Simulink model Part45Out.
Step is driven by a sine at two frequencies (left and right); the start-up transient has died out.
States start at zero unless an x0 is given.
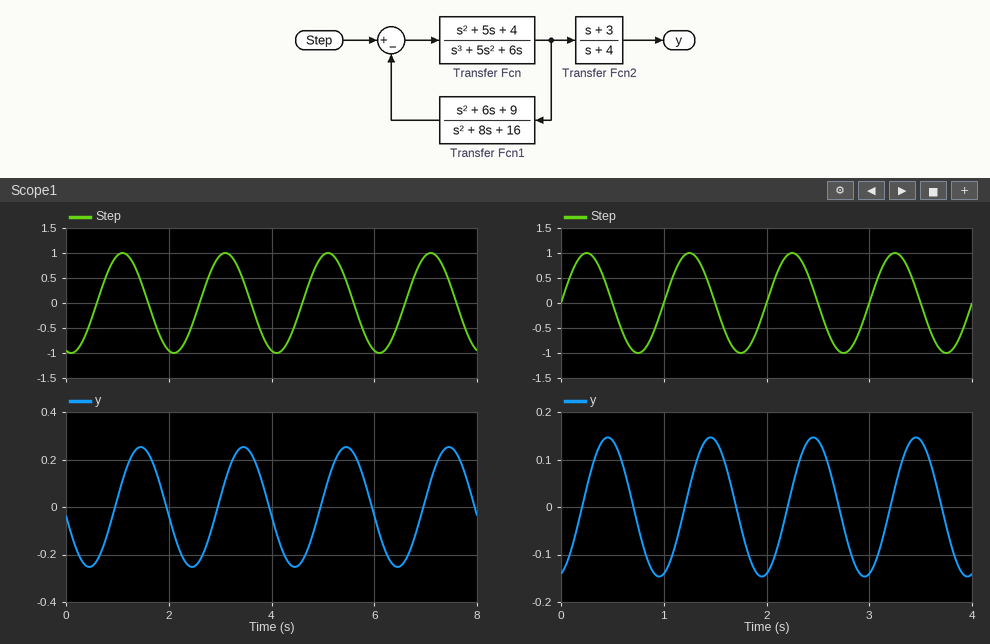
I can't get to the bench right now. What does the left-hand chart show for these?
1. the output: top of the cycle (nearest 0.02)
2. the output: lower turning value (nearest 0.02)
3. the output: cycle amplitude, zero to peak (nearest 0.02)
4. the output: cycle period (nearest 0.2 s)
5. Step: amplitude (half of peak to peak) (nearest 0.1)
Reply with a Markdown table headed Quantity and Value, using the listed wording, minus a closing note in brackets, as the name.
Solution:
| Quantity | Value |
|---|---|
| the output: top of the cycle | 0.26 |
| the output: lower turning value | -0.26 |
| the output: cycle amplitude, zero to peak | 0.26 |
| the output: cycle period | 2.0 s |
| Step: amplitude (half of peak to peak) | 1.0 |
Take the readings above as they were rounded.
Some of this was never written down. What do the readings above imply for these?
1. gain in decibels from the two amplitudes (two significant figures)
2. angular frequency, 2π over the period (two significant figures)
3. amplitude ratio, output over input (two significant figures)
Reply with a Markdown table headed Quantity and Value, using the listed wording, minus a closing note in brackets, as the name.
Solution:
| Quantity | Value |
|---|---|
| gain in decibels from the two amplitudes | -12 dB |
| angular frequency, 2π over the period | 3.1 rad/s |
| amplitude ratio, output over input | 0.26 |
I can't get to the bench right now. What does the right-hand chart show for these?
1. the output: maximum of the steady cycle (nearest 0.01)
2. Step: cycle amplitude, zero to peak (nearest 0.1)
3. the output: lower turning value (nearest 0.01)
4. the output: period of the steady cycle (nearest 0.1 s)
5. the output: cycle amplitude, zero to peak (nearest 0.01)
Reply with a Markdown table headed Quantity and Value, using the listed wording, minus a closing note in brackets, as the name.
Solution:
| Quantity | Value |
|---|---|
| the output: maximum of the steady cycle | 0.15 |
| Step: cycle amplitude, zero to peak | 1.0 |
| the output: lower turning value | -0.15 |
| the output: period of the steady cycle | 1.0 s |
| the output: cycle amplitude, zero to peak | 0.15 |
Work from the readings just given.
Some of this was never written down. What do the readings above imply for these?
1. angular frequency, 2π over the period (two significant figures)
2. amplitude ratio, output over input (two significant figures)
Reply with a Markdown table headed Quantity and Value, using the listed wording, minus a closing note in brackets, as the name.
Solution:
| Quantity | Value |
|---|---|
| angular frequency, 2π over the period | 6.3 rad/s |
| amplitude ratio, output over input | 0.15 |
